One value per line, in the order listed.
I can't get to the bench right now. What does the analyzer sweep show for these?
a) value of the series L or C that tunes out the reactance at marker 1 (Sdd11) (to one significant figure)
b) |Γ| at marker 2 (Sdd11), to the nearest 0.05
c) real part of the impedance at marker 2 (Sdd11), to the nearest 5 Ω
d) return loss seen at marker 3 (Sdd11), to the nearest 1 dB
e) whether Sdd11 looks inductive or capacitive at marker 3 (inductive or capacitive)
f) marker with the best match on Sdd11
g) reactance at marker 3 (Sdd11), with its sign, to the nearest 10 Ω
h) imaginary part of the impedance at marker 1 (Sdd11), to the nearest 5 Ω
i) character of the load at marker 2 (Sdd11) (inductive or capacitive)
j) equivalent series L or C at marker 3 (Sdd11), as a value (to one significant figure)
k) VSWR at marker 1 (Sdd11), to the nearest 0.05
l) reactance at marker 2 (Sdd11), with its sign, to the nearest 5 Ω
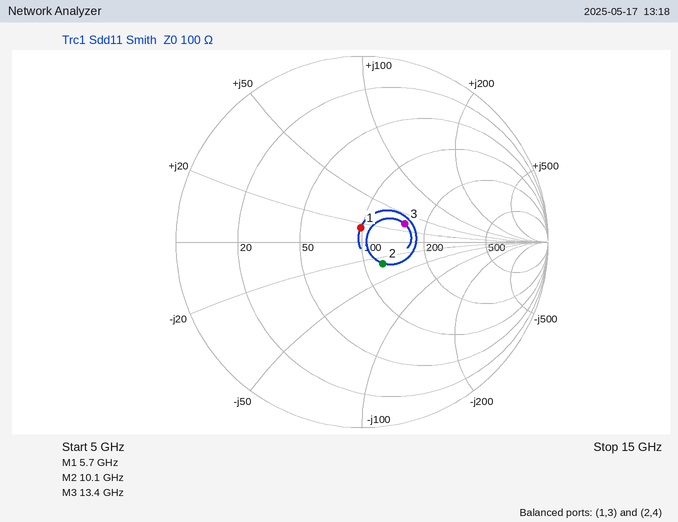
2 pF
0.15
120 Ω
12 dB
inductive
marker 1
+30 Ω
+15 Ω
capacitive
400 pH
1.15
-30 Ω
